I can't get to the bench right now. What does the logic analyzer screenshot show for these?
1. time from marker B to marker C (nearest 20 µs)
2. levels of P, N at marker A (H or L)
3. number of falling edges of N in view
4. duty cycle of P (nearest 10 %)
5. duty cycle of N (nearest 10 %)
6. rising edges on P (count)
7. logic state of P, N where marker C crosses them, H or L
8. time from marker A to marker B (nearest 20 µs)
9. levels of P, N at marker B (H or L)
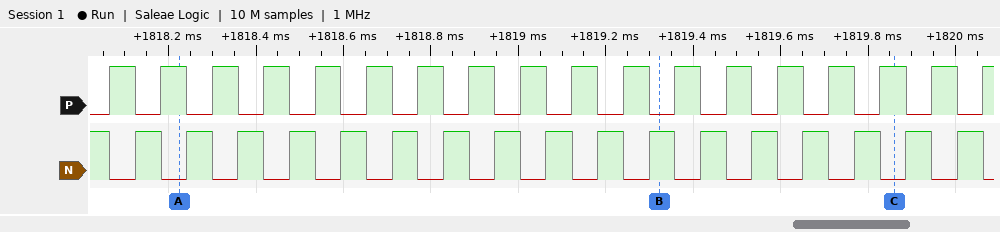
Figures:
540 µs
P=H, N=L
18
50 %
50 %
18
P=H, N=L
1100 µs
P=L, N=H
